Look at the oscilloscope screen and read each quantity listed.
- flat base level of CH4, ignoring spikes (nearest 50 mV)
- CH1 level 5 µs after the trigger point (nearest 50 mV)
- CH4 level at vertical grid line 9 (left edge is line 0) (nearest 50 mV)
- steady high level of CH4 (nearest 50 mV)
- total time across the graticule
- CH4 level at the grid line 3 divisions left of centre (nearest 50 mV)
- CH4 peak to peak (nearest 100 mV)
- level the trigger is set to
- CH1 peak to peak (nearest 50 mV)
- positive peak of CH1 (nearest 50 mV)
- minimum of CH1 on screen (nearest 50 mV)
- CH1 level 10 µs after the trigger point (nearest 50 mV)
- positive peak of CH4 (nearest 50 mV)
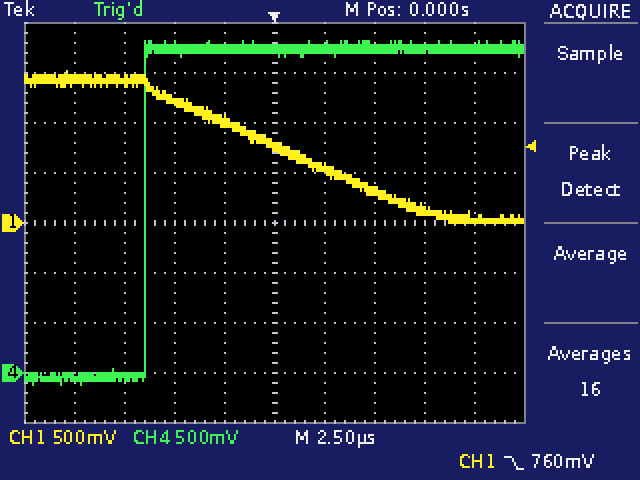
-50 mV
300 mV
3.25 V
3.25 V
25 µs
-50 mV
3.40 V
760 mV
1.50 V
1.50 V
0 mV
0 mV
3.30 V
